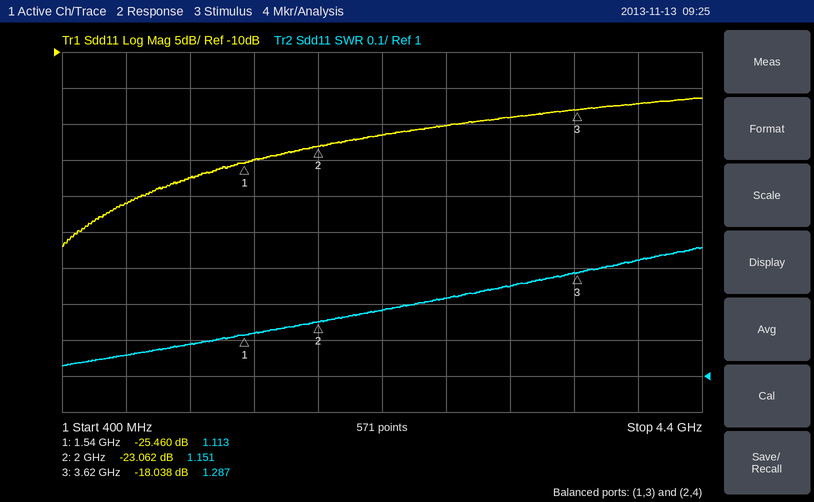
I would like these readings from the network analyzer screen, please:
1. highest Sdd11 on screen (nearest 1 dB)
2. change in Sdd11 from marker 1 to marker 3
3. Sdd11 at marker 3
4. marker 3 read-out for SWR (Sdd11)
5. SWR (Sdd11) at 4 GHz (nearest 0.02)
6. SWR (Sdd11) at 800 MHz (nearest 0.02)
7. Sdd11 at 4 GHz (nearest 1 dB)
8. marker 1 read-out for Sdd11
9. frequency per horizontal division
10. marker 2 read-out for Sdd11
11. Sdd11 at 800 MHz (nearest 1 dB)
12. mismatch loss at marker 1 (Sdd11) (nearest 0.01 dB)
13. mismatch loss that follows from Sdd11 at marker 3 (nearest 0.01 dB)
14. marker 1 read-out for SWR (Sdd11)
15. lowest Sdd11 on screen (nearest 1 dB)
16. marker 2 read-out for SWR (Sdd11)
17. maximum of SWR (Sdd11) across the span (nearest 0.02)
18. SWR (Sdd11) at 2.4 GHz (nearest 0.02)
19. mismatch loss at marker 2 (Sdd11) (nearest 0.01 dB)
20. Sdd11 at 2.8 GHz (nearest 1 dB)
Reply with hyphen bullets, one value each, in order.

- -16 dB
- 7.422 dB
- -18.038 dB
- 1.287
- 1.32
- 1.06
- -17 dB
- -25.460 dB
- 400 MHz
- -23.062 dB
- -31 dB
- 0.01 dB
- 0.07 dB
- 1.113
- -37 dB
- 1.151
- 1.36
- 1.18
- 0.02 dB
- -20 dB
